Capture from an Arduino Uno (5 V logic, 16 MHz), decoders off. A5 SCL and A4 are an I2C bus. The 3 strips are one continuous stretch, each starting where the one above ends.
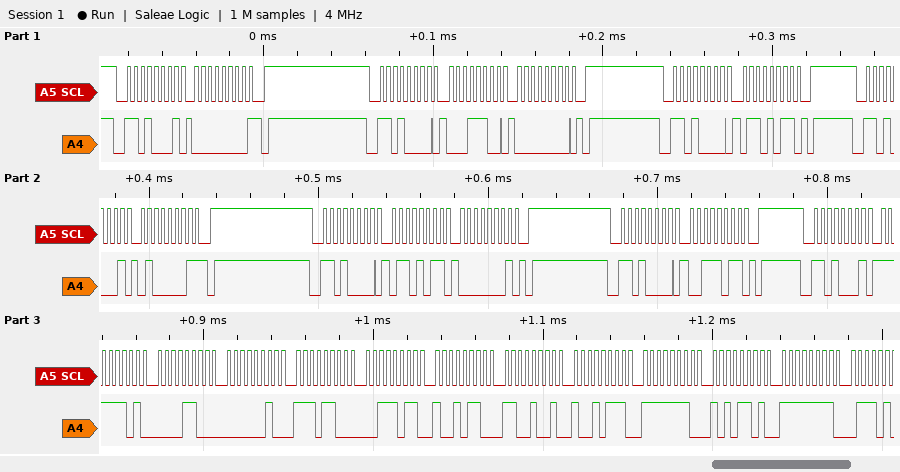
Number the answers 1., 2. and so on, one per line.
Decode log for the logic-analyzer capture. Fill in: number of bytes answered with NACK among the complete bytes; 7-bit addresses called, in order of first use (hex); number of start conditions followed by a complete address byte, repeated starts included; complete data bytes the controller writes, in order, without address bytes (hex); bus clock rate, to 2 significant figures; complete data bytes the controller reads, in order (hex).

1. 2
2. 0x68
3. 7
4. 1C 00 6B 6B 01 3B
5. 250 kHz
6. 00 41 FD 0C 02 EC 3B 96 C9 97 FE AD FF
